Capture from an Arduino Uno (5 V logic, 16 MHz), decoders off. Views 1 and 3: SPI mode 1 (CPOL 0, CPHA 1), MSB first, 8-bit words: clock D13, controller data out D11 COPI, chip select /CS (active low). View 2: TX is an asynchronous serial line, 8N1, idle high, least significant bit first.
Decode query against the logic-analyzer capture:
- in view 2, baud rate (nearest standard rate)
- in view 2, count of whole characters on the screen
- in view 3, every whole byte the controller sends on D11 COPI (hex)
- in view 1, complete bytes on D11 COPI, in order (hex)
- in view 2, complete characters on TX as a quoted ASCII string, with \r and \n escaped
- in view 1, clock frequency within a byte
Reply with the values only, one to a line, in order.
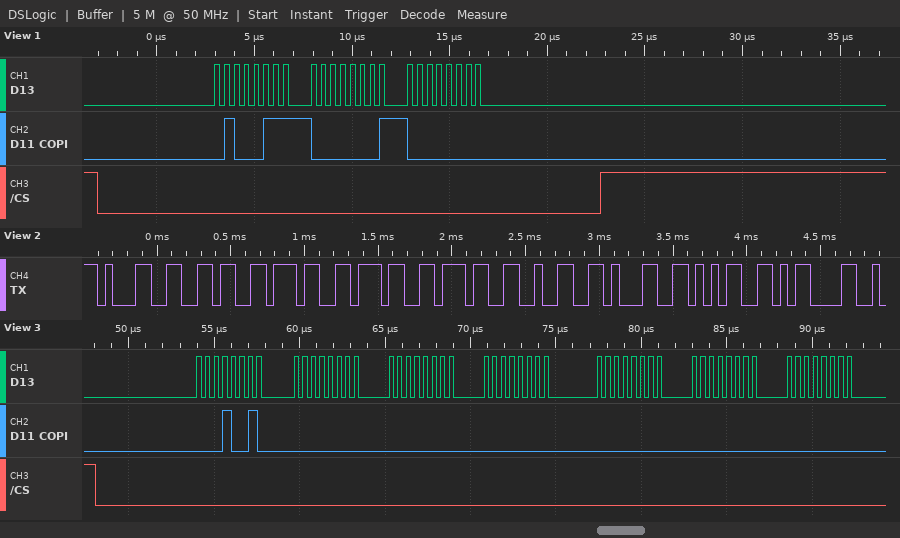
19200 baud
9
12 00 00 00 00 00 00
47 01 00
"16777215\r"
2 MHz
